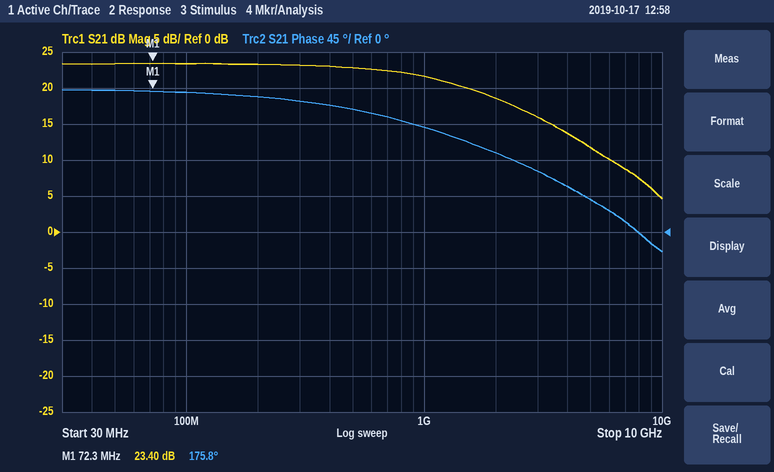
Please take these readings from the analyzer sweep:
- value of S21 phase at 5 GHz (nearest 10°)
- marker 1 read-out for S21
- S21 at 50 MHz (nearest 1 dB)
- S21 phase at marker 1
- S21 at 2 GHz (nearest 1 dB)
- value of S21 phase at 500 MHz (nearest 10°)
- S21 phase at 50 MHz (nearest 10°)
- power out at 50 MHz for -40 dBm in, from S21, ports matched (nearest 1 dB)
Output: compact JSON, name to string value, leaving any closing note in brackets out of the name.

{"value of S21 phase at 5 GHz": "40°", "marker 1 read-out for S21": "23.40 dB", "S21 at 50 MHz": "23 dB", "S21 phase at marker 1": "175.8°", "S21 at 2 GHz": "19 dB", "value of S21 phase at 500 MHz": "150°", "S21 phase at 50 MHz": "180°", "power out at 50 MHz for -40 dBm in, from S21, ports matched": "-17 dBm"}
